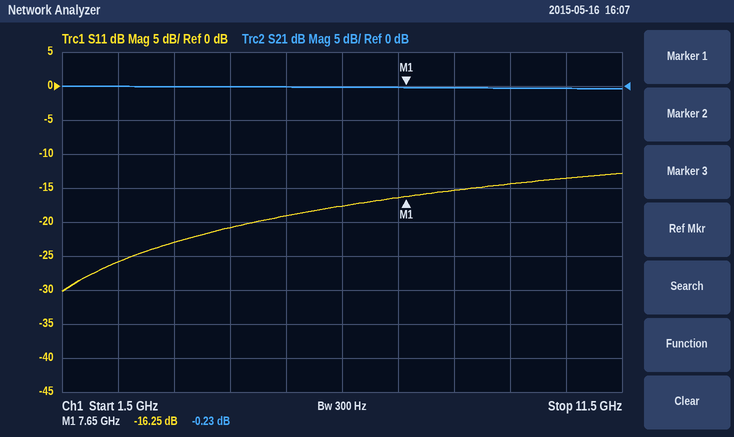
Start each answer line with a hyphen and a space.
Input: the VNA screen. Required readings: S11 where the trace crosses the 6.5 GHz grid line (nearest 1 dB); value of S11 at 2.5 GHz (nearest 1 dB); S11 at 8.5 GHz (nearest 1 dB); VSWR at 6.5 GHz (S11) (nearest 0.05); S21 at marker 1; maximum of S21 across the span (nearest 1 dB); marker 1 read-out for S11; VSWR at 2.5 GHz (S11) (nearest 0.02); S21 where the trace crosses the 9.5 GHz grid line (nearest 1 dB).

- -18 dB
- -26 dB
- -15 dB
- 1.30
- -0.23 dB
- 0 dB
- -16.25 dB
- 1.10
- 0 dB
